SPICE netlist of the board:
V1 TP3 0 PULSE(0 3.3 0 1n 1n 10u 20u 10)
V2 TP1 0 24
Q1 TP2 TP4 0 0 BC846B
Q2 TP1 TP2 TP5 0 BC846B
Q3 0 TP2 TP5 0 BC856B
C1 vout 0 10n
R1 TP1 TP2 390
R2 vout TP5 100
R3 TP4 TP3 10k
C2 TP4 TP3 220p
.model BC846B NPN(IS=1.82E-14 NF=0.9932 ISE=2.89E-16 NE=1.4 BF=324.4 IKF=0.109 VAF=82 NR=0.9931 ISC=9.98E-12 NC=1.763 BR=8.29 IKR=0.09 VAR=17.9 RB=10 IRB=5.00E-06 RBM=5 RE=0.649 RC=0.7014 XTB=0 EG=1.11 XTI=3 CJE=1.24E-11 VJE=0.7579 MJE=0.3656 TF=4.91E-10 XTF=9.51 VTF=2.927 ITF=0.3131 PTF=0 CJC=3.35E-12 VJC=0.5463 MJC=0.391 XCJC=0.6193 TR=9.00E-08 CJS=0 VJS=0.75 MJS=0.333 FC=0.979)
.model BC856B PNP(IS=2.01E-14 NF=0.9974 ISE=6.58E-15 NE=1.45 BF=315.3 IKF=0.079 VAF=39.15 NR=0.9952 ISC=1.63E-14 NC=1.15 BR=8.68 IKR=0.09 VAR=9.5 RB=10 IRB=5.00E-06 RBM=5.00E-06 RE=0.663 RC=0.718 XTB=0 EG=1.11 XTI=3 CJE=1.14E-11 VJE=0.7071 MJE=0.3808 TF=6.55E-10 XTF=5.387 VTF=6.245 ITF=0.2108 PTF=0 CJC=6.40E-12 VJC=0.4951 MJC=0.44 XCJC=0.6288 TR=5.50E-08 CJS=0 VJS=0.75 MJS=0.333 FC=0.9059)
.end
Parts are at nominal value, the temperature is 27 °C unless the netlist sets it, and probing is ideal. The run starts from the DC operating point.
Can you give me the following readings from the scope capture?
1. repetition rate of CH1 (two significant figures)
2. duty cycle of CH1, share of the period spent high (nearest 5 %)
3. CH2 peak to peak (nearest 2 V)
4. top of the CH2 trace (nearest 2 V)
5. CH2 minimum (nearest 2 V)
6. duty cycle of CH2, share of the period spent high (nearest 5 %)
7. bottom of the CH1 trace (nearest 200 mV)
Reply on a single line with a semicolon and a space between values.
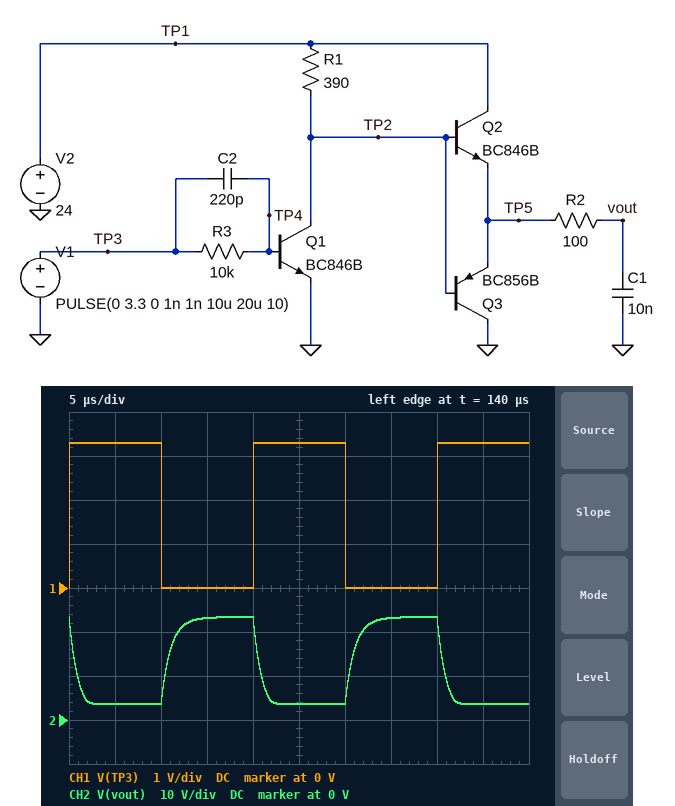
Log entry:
50 kHz; 50 %; 20 V; 24 V; 4 V; 50 %; 0 V
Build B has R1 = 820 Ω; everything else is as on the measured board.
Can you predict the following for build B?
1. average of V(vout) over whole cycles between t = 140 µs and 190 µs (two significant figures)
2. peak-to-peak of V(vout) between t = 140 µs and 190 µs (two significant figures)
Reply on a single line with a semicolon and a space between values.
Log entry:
12 V; 23 V
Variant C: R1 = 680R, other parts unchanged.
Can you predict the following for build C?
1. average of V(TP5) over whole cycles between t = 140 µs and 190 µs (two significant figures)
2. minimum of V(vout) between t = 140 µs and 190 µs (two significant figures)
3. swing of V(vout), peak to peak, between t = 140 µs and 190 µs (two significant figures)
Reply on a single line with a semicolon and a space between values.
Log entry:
12 V; 750 mV; 23 V
